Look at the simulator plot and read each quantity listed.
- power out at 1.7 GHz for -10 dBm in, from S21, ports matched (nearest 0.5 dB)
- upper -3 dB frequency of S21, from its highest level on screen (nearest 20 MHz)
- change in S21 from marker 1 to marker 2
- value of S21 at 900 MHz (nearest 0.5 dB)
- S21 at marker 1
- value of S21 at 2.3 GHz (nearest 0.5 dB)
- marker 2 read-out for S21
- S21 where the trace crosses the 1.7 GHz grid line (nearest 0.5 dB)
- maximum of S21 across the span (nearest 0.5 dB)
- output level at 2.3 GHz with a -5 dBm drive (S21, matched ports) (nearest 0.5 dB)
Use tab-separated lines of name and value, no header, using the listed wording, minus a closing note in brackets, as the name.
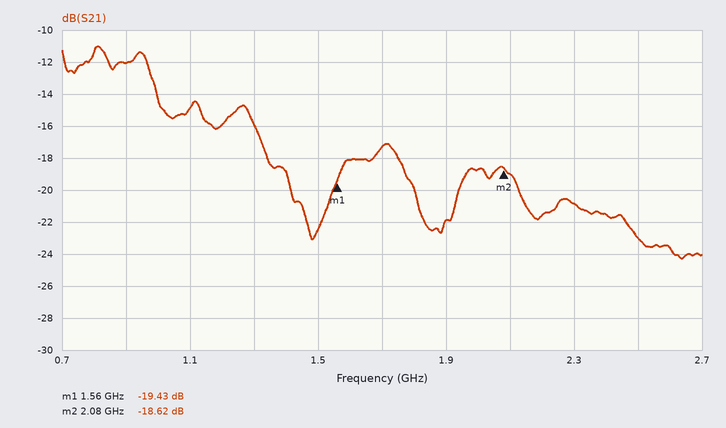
power out at 1.7 GHz for -10 dBm in, from S21, ports matched	-27.5 dBm
upper -3 dB frequency of S21, from its highest level on screen	1.00 GHz
change in S21 from marker 1 to marker 2	0.81 dB
value of S21 at 900 MHz	-12.0 dB
S21 at marker 1	-19.43 dB
value of S21 at 2.3 GHz	-21.0 dB
marker 2 read-out for S21	-18.62 dB
S21 where the trace crosses the 1.7 GHz grid line	-17.5 dB
maximum of S21 across the span	-11.0 dB
output level at 2.3 GHz with a -5 dBm drive (S21, matched ports)	-26.0 dBm
